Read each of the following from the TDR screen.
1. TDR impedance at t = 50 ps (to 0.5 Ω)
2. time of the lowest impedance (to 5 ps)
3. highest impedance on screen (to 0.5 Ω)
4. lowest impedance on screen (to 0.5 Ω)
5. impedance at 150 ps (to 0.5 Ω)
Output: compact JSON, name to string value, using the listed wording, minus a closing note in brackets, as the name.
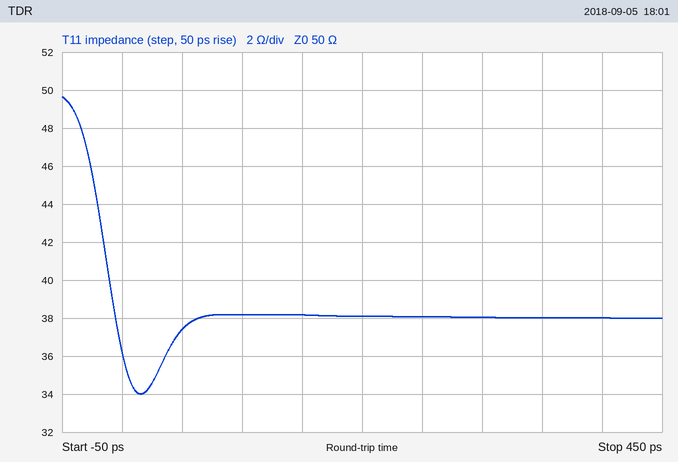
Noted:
{"TDR impedance at t = 50 ps": "37.5 Ω", "time of the lowest impedance": "15 ps", "highest impedance on screen": "49.5 Ω", "lowest impedance on screen": "34.0 Ω", "impedance at 150 ps": "38.0 Ω"}
